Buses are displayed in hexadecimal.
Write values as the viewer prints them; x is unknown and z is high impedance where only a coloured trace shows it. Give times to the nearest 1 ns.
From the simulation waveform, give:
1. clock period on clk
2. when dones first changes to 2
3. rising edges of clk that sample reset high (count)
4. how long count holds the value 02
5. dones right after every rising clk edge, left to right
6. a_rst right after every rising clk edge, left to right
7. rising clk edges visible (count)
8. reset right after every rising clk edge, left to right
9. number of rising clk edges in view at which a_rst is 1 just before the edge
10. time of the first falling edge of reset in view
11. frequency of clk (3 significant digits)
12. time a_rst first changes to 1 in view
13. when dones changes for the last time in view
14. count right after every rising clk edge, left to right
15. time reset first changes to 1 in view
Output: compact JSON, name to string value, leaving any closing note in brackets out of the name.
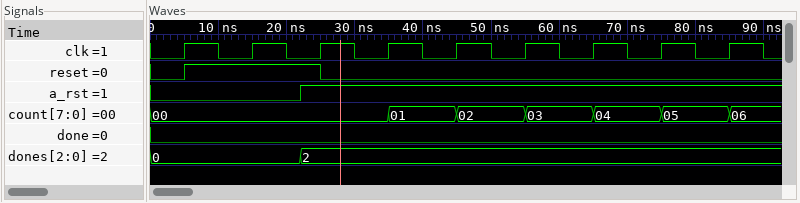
{"clock period on clk": "10 ns", "when dones first changes to 2": "22 ns", "rising edges of clk that sample reset high": "2", "how long count holds the value 02": "10 ns", "dones right after every rising clk edge, left to right": "0, 0, 2, 2, 2, 2, 2, 2, 2", "a_rst right after every rising clk edge, left to right": "0 0 1 1 1 1 1 1 1", "rising clk edges visible": "9", "reset right after every rising clk edge, left to right": "1 1 0 0 0 0 0 0 0", "number of rising clk edges in view at which a_rst is 1 just before the edge": "7", "time of the first falling edge of reset in view": "25 ns", "frequency of clk": "100 MHz", "time a_rst first changes to 1 in view": "22 ns", "when dones changes for the last time in view": "22 ns", "count right after every rising clk edge, left to right": "00, 00, 00, 01, 02, 03, 04, 05, 06", "time reset first changes to 1 in view": "5 ns"}
